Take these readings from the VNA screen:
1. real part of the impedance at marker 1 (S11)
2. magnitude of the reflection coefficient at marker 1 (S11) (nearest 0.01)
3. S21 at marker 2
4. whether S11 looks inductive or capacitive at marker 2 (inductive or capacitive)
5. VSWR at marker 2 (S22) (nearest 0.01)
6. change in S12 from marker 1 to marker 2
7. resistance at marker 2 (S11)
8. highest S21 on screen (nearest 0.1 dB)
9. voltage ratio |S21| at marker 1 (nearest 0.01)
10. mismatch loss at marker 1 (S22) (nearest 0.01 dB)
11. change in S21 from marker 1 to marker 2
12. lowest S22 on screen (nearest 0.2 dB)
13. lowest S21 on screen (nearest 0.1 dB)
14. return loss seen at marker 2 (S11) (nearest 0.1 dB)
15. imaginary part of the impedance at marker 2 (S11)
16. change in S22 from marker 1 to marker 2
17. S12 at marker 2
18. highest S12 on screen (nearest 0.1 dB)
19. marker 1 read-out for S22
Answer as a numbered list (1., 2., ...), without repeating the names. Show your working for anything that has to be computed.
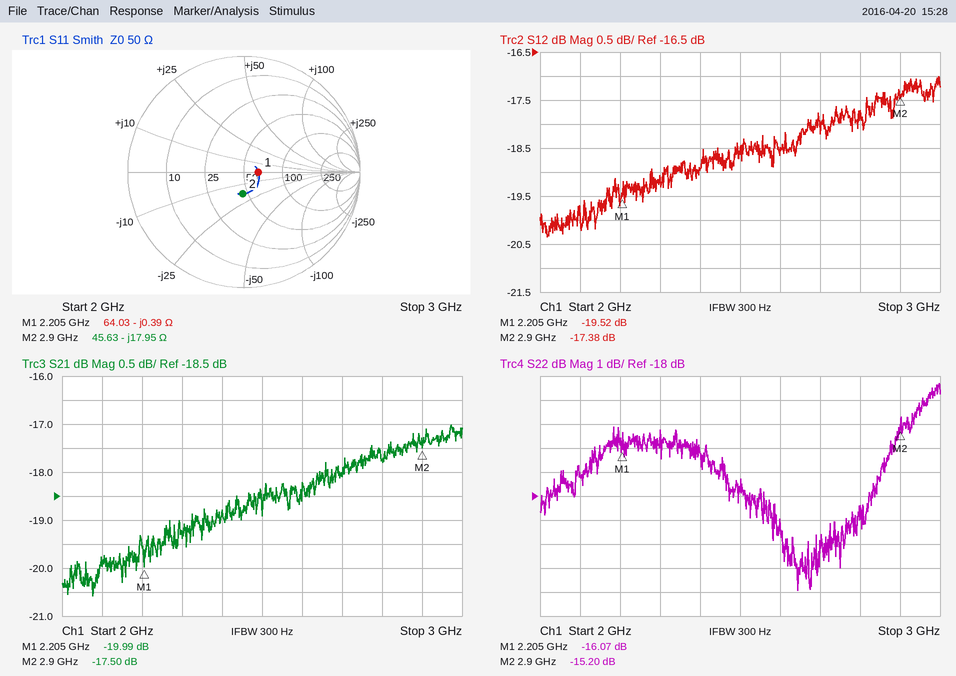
1. 64.03 Ω
2. 0.12
3. -17.50 dB
4. capacitive
5. (1 + 0.1738)/(1 − 0.1738) ≈ 1.42
6. -17.38 − (-19.52) = 2.14 dB
7. 45.63 Ω
8. -17.0 dB
9. 10^(-19.99/20) ≈ 0.10
10. −10 log10(1 − 10^(-16.07/10)) ≈ 0.11 dB
11. -17.5 − (-19.99) = 2.49 dB
12. -22.0 dB
13. -20.6 dB
14. 14.4 dB
15. -17.95 Ω
16. -15.2 − (-16.07) = 0.87 dB
17. -17.38 dB
18. -17.0 dB
19. -16.07 dB
